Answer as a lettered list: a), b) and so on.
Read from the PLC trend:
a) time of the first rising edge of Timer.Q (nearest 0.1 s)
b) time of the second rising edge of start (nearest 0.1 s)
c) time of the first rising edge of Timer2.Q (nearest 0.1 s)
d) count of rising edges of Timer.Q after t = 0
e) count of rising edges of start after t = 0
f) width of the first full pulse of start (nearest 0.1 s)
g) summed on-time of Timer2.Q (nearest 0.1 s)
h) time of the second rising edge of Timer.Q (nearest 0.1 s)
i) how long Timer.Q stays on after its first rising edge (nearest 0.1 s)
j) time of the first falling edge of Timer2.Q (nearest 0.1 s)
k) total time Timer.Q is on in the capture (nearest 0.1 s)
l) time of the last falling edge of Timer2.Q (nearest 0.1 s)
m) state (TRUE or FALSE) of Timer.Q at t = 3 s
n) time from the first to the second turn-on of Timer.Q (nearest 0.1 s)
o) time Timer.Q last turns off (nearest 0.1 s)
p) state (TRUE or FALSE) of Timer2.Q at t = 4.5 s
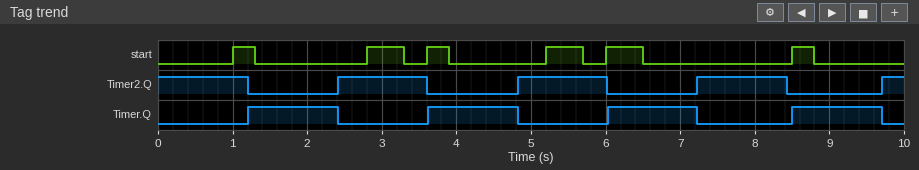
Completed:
a) 1.2 s
b) 2.8 s
c) 2.4 s
d) 4
e) 6
f) 0.3 s
g) 5.1 s
h) 3.6 s
i) 1.2 s
j) 1.2 s
k) 4.8 s
l) 8.4 s
m) FALSE
n) 2.4 s
o) 9.7 s
p) FALSE
